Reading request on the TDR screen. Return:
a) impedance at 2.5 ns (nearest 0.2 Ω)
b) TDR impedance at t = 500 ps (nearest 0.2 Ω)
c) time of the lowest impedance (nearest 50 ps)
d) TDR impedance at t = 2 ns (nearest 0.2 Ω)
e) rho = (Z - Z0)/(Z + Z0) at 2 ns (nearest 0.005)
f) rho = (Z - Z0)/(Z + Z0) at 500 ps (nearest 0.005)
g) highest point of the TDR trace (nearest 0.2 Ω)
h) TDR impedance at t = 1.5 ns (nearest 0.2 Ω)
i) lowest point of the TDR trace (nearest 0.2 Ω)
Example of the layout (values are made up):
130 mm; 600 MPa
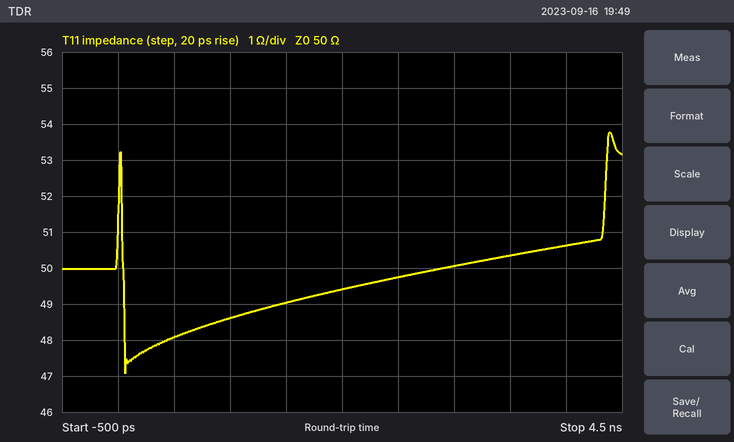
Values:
49.8 Ω; 48.0 Ω; 50 ps; 49.4 Ω; -0.005; -0.020; 53.8 Ω; 49.0 Ω; 47.0 Ω
